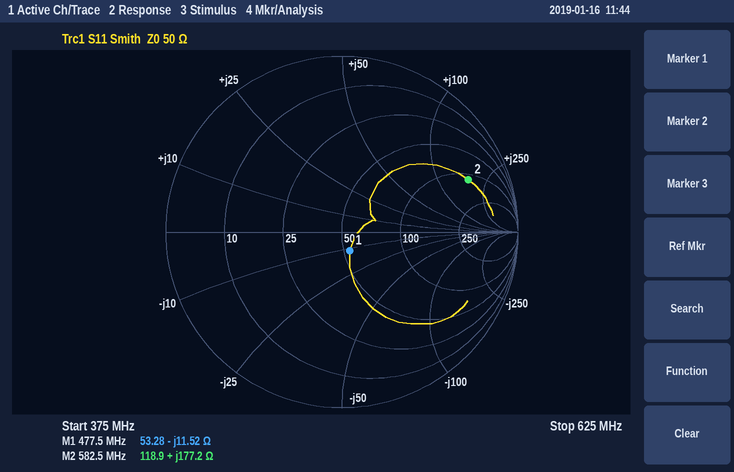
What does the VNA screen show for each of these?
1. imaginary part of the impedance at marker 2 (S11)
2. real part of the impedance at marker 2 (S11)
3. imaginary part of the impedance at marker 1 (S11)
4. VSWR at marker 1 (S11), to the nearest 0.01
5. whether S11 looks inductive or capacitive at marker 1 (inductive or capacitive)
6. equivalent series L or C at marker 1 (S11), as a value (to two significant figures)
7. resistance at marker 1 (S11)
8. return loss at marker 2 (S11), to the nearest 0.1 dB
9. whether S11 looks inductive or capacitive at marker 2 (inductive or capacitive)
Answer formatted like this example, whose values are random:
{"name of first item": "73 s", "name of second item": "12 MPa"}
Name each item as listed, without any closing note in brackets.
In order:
{"imaginary part of the impedance at marker 2": "+177.2 Ω", "real part of the impedance at marker 2": "118.9 Ω", "imaginary part of the impedance at marker 1": "-11.52 Ω", "VSWR at marker 1 (S11), to the nearest 0.01": "1.26", "whether S11 looks inductive or capacitive at marker 1": "capacitive", "equivalent series L or C at marker 1 (S11), as a value": "29 pF", "resistance at marker 1": "53.28 Ω", "return loss at marker 2 (S11), to the nearest 0.1 dB": "2.2 dB", "whether S11 looks inductive or capacitive at marker 2": "inductive"}
